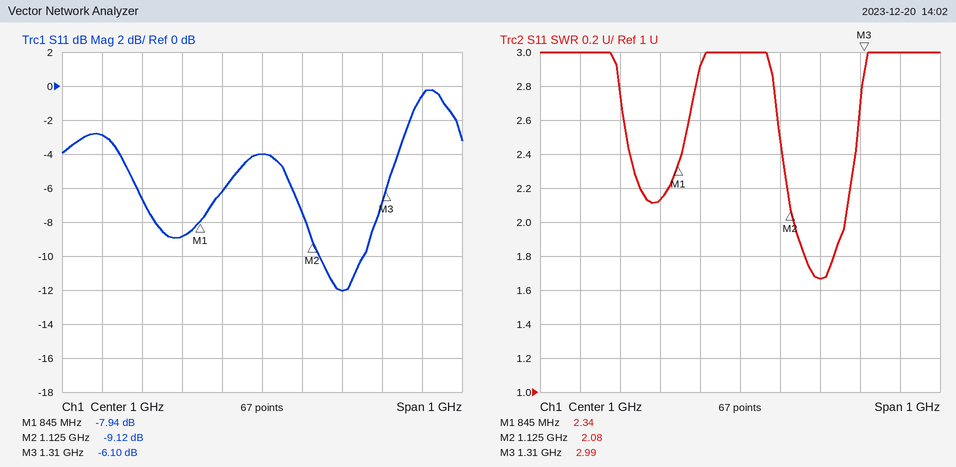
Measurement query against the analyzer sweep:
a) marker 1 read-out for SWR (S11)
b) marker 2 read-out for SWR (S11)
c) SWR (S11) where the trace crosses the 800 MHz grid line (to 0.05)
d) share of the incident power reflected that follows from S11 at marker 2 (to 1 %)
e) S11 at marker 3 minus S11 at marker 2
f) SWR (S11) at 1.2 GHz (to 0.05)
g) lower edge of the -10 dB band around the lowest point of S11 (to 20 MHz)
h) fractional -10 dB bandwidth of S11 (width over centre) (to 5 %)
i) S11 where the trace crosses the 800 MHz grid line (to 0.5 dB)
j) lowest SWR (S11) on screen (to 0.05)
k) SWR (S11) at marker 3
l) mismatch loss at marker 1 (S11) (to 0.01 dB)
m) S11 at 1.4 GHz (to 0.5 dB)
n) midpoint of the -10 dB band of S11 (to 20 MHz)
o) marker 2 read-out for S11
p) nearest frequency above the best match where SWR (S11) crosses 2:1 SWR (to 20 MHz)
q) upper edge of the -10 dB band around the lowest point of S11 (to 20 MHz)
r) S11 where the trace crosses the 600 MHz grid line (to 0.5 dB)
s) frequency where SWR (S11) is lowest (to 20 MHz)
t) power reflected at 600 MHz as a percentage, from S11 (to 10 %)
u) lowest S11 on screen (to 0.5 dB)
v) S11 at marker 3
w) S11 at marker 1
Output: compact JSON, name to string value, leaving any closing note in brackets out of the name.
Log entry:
{"marker 1 read-out for SWR": "2.34", "marker 2 read-out for SWR": "2.08", "SWR (S11) where the trace crosses the 800 MHz grid line": "2.15", "share of the incident power reflected that follows from S11 at marker 2": "12 %", "S11 at marker 3 minus S11 at marker 2": "3.02 dB", "SWR (S11) at 1.2 GHz": "1.65", "lower edge of the -10 dB band around the lowest point of S11": "1.14 GHz", "fractional -10 dB bandwidth of S11 (width over centre)": "10 %", "S11 where the trace crosses the 800 MHz grid line": "-9.0 dB", "lowest SWR (S11) on screen": "1.65", "SWR (S11) at marker 3": "2.99", "mismatch loss at marker 1 (S11)": "0.76 dB", "S11 at 1.4 GHz": "-0.5 dB", "midpoint of the -10 dB band of S11": "1.20 GHz", "marker 2 read-out for S11": "-9.12 dB", "nearest frequency above the best match where SWR (S11) crosses 2:1 SWR": "1.26 GHz", "upper edge of the -10 dB band around the lowest point of S11": "1.26 GHz", "S11 where the trace crosses the 600 MHz grid line": "-3.0 dB", "frequency where SWR (S11) is lowest": "1.20 GHz", "power reflected at 600 MHz as a percentage, from S11": "50 %", "lowest S11 on screen": "-12.0 dB", "S11 at marker 3": "-6.10 dB", "S11 at marker 1": "-7.94 dB"}
